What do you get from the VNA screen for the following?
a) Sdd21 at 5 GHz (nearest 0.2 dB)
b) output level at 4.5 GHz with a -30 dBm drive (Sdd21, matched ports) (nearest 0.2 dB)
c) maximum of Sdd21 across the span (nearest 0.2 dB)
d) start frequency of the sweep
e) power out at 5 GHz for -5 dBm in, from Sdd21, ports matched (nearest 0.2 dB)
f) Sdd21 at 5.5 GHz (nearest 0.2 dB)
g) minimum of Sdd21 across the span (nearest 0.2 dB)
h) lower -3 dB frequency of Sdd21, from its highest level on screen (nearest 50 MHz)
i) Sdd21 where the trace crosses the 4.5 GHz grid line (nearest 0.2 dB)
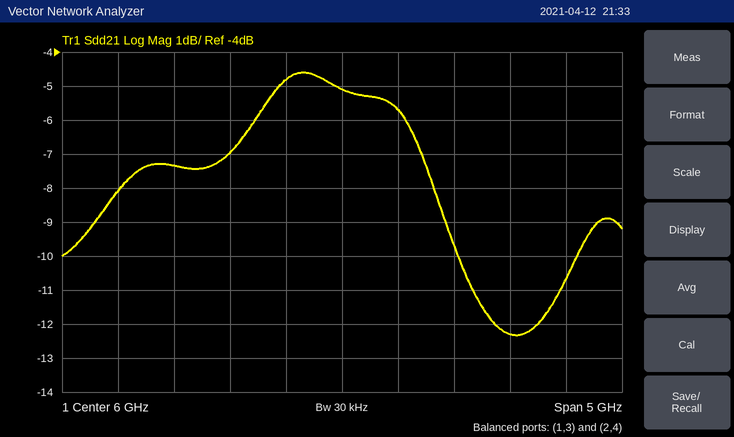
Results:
-7.0 dB
-37.4 dBm
-4.6 dB
3.5 GHz
-12.0 dBm
-4.8 dB
-12.4 dB
4.15 GHz
-7.4 dB
